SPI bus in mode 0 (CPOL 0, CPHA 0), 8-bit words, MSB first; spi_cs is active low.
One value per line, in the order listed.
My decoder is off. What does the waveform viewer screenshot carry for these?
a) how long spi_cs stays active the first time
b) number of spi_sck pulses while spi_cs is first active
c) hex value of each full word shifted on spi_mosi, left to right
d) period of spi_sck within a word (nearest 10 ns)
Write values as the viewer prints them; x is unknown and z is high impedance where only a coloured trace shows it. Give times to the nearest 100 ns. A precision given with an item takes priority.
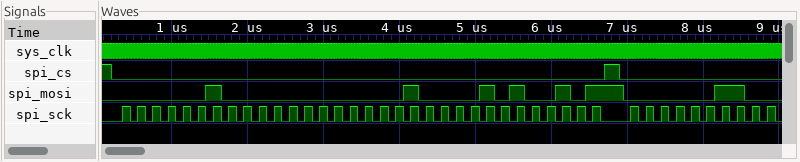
6500 ns
32
02, 00, 10, A5, 03
200 ns
